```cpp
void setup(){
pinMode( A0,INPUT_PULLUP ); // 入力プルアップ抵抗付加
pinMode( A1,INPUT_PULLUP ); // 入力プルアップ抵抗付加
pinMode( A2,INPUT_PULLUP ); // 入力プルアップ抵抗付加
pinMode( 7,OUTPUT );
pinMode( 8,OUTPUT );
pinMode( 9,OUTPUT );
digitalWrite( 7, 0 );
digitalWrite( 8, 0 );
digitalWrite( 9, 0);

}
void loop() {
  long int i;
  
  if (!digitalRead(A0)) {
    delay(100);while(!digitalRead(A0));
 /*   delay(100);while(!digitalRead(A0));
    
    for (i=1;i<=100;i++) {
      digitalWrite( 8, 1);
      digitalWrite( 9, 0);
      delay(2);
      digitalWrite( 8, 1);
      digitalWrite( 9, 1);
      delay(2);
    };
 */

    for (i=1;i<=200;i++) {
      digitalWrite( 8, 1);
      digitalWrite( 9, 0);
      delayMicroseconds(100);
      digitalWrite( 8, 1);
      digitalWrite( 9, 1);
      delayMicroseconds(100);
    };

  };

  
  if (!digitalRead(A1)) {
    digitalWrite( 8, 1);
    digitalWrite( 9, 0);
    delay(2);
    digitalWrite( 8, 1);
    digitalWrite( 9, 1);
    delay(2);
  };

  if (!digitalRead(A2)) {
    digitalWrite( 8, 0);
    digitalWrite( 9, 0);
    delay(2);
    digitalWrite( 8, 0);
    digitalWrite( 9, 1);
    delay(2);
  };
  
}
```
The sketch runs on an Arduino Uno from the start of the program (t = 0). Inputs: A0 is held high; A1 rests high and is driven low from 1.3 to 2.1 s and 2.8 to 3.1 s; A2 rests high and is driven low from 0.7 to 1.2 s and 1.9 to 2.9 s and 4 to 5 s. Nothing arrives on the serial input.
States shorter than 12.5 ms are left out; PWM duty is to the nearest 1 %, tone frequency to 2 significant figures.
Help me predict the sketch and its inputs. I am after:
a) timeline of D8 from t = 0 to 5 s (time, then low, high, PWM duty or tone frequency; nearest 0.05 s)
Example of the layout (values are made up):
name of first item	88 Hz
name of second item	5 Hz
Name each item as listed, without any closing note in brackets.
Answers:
timeline of D8 from t = 0 to 5 s	0 s low; 1.3 s high; 1.9 s tone 120 Hz; 2.1 s low; 2.8 s tone 120 Hz; 2.9 s high; 4 s low
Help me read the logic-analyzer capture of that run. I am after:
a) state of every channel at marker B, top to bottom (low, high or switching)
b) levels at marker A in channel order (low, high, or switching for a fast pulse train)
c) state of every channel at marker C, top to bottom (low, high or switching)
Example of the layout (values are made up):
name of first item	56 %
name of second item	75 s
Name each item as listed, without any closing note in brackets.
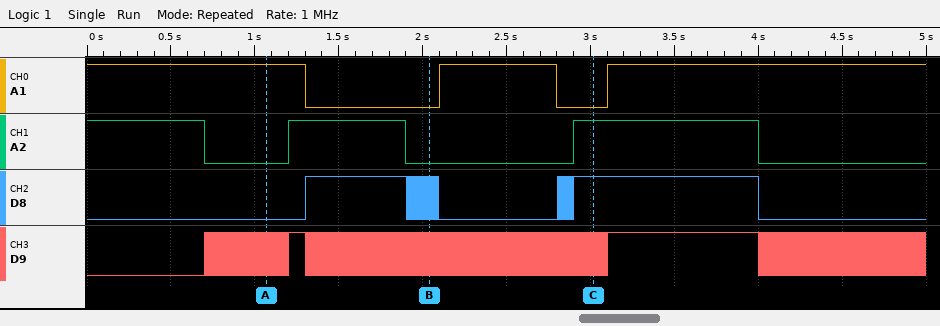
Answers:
state of every channel at marker B, top to bottom	A1 low, A2 low, D8 switching, D9 switching
levels at marker A in channel order	A1 high, A2 low, D8 low, D9 switching
state of every channel at marker C, top to bottom	A1 low, A2 high, D8 high, D9 switching
